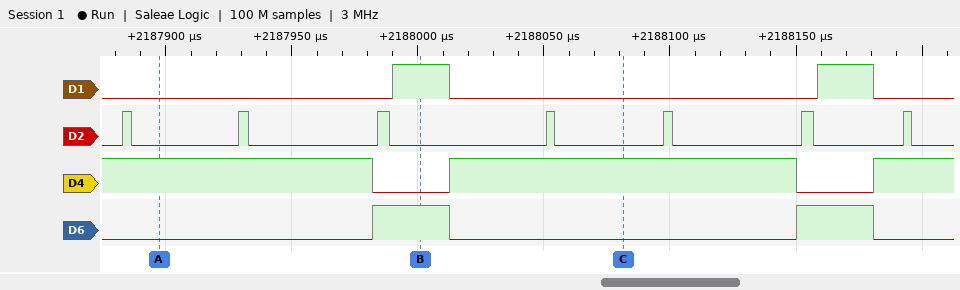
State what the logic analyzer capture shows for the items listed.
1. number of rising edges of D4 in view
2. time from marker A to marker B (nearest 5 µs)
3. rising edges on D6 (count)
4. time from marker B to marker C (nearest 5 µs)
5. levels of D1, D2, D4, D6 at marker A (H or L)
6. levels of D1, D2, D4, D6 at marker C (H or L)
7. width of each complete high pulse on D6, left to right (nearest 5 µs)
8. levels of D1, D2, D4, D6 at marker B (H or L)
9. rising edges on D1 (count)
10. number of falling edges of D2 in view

2
105 µs
2
80 µs
D1=L, D2=L, D4=H, D6=L
D1=L, D2=L, D4=H, D6=L
30 µs, 30 µs
D1=H, D2=L, D4=L, D6=H
2
7
